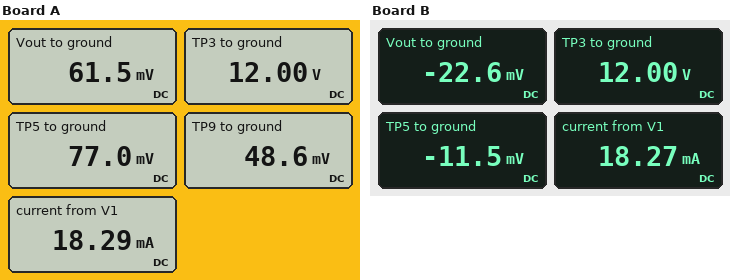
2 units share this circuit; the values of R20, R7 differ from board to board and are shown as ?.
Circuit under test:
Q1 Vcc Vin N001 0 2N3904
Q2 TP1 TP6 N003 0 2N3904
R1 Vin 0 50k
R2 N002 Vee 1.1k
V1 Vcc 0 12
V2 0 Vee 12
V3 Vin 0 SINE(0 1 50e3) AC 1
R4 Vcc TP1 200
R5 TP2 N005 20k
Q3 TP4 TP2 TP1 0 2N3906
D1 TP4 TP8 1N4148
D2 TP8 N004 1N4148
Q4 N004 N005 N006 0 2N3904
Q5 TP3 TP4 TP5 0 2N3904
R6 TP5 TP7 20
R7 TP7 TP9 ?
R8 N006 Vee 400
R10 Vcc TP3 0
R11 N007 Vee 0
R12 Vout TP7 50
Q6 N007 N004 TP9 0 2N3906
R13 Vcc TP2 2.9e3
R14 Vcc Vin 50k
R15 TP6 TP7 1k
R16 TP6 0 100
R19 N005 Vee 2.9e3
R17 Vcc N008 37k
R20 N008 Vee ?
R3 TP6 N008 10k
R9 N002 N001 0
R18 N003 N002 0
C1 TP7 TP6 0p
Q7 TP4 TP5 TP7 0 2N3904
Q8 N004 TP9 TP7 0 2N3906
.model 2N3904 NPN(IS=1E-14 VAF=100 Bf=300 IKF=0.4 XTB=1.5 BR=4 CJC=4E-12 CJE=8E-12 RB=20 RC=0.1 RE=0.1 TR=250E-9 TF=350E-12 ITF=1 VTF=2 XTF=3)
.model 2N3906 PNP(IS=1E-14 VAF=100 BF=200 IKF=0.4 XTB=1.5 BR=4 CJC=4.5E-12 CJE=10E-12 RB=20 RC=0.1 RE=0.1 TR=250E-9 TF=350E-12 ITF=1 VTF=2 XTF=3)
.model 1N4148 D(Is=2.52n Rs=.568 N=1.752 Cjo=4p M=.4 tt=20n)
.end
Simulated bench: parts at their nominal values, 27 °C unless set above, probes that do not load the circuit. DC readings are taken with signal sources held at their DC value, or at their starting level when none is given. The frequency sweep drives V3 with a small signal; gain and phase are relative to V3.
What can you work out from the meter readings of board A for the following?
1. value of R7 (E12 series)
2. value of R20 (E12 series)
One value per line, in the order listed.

18 Ω
27 kΩ
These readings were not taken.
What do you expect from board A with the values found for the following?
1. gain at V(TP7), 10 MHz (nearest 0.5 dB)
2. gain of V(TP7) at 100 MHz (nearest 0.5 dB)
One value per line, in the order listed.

21.0 dB
3.0 dB
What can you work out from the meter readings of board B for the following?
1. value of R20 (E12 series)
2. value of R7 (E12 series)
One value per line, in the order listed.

39 kΩ
56 Ω
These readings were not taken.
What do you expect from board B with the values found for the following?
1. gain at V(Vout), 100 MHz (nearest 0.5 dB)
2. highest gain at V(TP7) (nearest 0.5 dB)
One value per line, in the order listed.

3.0 dB
21.0 dB
